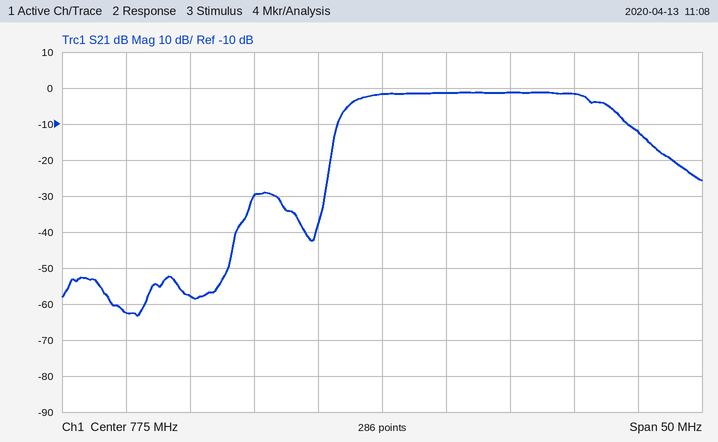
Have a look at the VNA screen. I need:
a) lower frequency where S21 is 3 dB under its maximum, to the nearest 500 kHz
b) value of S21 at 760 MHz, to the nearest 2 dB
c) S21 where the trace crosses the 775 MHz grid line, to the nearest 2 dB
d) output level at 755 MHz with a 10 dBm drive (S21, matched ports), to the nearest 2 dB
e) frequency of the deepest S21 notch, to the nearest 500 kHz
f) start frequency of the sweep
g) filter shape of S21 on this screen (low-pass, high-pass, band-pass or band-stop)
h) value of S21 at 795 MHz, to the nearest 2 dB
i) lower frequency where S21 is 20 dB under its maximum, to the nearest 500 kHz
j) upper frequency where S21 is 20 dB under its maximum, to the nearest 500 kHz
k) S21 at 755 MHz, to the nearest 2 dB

772.5 MHz
-58 dB
-2 dB
-52 dBm
756.0 MHz
750 MHz
band-pass
-12 dB
771.0 MHz
798.0 MHz
-62 dB
